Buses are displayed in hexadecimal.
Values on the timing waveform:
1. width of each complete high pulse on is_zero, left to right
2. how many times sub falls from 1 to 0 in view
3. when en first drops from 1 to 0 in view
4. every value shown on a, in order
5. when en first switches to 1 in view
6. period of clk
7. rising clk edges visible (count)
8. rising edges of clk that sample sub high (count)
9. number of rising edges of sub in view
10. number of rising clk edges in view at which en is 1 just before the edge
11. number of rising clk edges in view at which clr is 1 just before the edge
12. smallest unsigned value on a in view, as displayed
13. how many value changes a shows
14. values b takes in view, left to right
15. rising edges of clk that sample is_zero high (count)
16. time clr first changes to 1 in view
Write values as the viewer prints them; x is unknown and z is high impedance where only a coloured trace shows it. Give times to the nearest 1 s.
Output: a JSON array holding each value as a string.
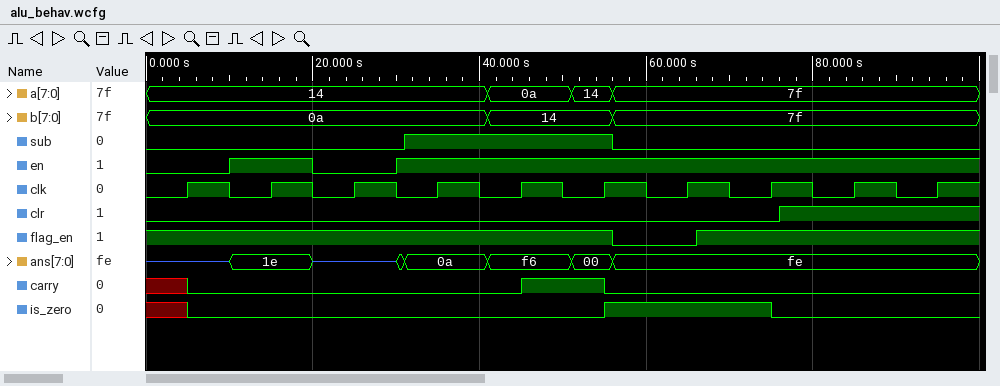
["20 s", "1", "20 s", "14, 0a, 14, 7f", "10 s", "10 s", "10", "3", "1", "8", "2", "0a", "3", "0a, 14, 7f", "2", "76 s"]
